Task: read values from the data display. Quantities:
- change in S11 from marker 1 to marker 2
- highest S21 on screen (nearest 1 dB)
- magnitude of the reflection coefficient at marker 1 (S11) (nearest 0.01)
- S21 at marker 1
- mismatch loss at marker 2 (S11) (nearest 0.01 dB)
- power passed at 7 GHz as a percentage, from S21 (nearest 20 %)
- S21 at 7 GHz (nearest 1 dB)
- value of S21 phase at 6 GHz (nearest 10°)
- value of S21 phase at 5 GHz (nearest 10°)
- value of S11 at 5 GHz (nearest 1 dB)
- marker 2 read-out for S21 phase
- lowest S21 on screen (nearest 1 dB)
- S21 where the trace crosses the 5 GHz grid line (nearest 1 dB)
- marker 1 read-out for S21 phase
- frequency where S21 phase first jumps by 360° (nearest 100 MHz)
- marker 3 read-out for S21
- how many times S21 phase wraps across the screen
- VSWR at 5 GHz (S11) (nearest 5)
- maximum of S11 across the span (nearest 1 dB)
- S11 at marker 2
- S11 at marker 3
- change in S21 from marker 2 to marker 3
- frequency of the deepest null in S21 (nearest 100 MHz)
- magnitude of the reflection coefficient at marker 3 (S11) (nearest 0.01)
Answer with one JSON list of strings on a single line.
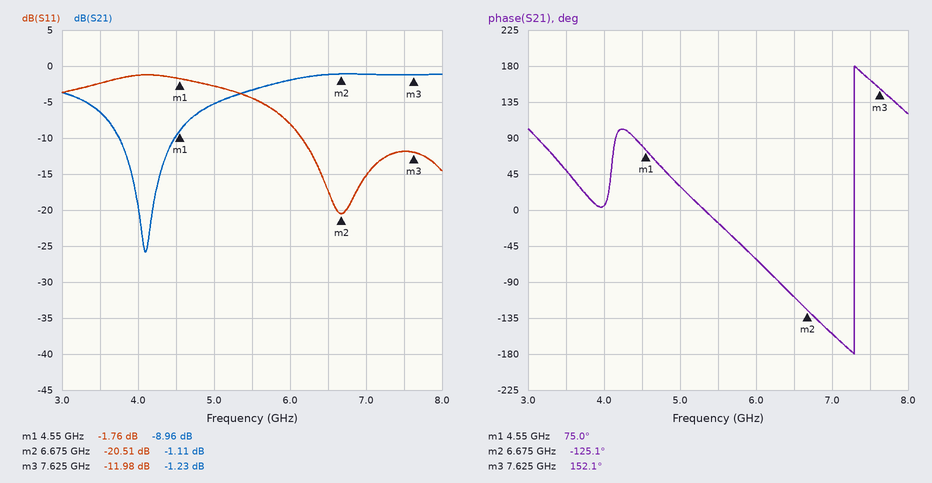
["-18.75 dB", "-1 dB", "0.82", "-8.96 dB", "0.04 dB", "80 %", "-1 dB", "-60°", "30°", "-3 dB", "-125.1°", "-26 dB", "-5 dB", "75.0°", "7.3 GHz", "-1.23 dB", "1", "5", "-1 dB", "-20.51 dB", "-11.98 dB", "-0.12 dB", "4.1 GHz", "0.25"]
